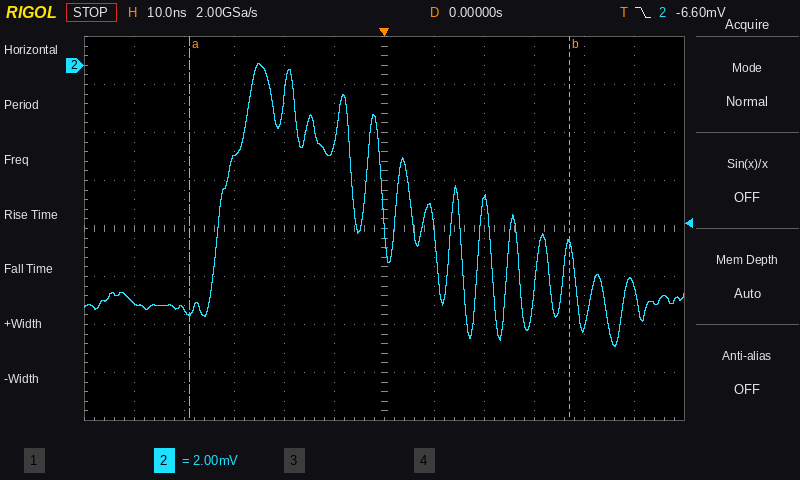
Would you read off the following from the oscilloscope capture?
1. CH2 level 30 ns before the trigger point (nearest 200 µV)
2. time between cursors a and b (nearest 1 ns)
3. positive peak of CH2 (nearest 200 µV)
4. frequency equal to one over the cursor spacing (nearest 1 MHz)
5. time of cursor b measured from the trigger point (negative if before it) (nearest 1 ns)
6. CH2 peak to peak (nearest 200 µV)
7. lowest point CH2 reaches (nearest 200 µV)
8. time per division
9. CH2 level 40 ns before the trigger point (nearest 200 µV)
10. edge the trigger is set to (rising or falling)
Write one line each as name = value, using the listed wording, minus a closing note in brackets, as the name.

CH2 level 30 ns before the trigger point = -3.8 mV
time between cursors a and b = 76 ns
positive peak of CH2 = 0.0 mV
frequency equal to one over the cursor spacing = 13 MHz
time of cursor b measured from the trigger point (negative if before it) = +37 ns
CH2 peak to peak = 11.8 mV
lowest point CH2 reaches = -11.8 mV
time per division = 10 ns
CH2 level 40 ns before the trigger point = -10.2 mV
edge the trigger is set to = falling
